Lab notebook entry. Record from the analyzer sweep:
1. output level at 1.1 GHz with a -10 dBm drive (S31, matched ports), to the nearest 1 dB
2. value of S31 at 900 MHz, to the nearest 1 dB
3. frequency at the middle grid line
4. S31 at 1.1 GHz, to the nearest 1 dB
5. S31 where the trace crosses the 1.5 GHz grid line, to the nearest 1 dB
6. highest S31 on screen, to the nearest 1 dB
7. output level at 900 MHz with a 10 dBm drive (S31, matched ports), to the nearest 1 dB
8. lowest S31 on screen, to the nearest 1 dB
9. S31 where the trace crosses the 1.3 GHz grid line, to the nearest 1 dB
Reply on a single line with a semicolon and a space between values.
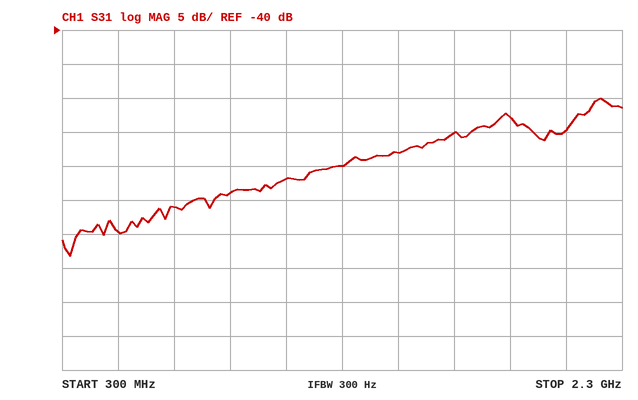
-72 dBm; -64 dB; 1.3 GHz; -62 dB; -58 dB; -50 dB; -54 dBm; -73 dB; -60 dB
